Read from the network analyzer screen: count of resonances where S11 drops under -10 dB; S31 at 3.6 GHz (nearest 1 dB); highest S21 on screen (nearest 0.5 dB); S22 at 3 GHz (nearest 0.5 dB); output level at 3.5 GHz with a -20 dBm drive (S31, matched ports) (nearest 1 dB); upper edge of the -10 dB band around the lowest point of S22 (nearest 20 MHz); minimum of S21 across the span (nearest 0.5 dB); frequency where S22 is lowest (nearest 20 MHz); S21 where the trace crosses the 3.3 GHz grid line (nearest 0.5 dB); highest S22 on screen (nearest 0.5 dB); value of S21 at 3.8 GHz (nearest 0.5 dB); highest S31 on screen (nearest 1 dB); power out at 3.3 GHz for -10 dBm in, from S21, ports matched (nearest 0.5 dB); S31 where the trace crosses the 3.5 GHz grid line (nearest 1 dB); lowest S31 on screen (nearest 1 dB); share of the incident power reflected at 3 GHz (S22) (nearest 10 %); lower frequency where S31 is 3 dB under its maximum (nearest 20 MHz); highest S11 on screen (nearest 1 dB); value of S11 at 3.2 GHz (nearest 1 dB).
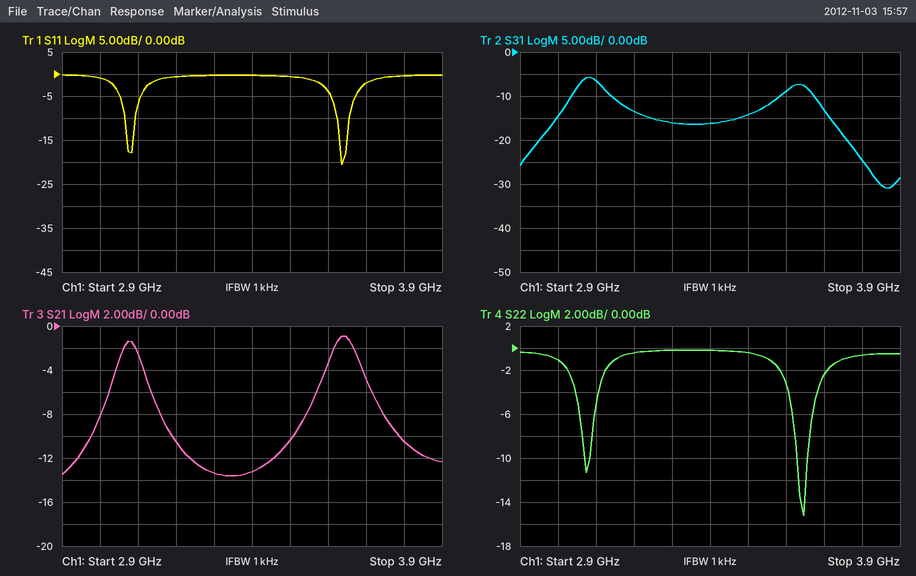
2
-9 dB
-1.0 dB
-1.0 dB
-34 dBm
3.66 GHz
-13.5 dB
3.64 GHz
-13.5 dB
0.0 dB
-10.5 dB
-6 dB
-23.5 dBm
-14 dB
-31 dB
80 %
3.04 GHz
0 dB
-1 dB
